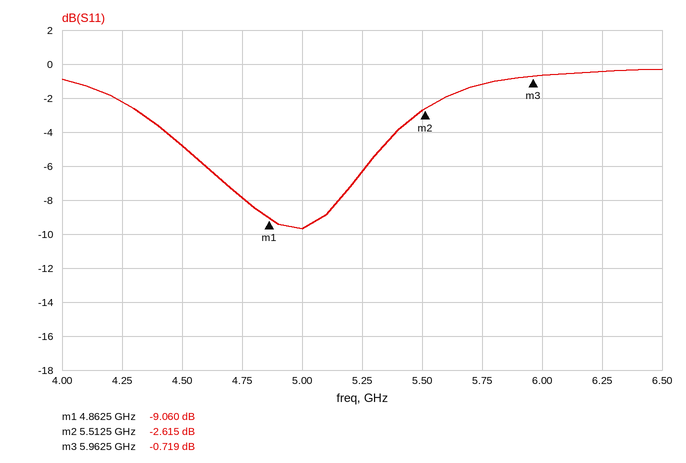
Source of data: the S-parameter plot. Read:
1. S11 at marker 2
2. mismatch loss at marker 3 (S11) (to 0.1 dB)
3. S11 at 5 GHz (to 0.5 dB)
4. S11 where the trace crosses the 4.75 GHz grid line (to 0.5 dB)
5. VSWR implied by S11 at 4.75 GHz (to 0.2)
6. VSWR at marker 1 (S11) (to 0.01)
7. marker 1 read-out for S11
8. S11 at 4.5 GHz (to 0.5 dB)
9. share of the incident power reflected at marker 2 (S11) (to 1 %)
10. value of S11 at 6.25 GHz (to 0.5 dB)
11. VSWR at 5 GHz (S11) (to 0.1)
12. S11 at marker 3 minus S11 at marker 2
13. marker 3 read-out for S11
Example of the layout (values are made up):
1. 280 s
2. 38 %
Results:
1. -2.615 dB
2. 8.2 dB
3. -9.5 dB
4. -8.0 dB
5. 2.4
6. 2.09
7. -9.060 dB
8. -5.0 dB
9. 55 %
10. -0.5 dB
11. 2.0
12. 1.896 dB
13. -0.719 dB
